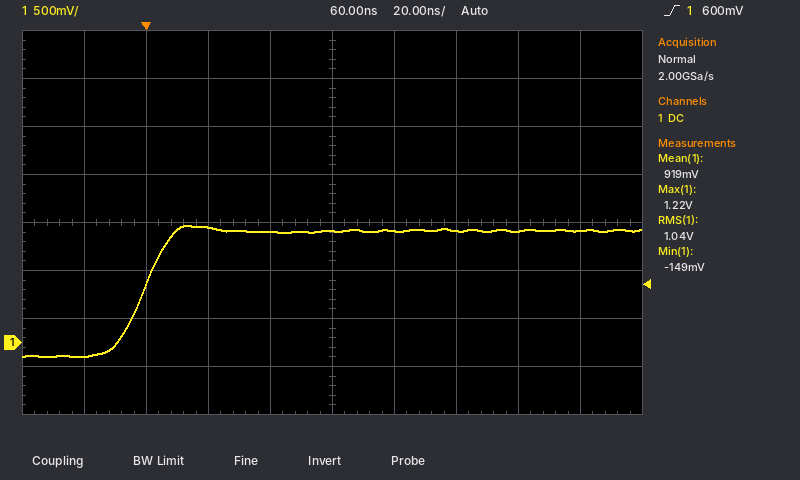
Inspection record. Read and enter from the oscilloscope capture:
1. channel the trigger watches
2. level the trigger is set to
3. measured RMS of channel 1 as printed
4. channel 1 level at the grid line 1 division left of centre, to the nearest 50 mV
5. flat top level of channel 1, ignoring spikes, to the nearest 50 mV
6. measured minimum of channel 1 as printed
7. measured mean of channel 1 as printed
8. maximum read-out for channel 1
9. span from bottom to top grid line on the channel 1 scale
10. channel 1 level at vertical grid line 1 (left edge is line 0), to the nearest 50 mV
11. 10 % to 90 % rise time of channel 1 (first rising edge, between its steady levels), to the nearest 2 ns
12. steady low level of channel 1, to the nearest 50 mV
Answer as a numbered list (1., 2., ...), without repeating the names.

1. channel 1
2. 600 mV
3. 1.04 V
4. 1.15 V
5. 1.15 V
6. -149 mV
7. 919 mV
8. 1.22 V
9. 4 V
10. -150 mV
11. 16 ns
12. -150 mV
